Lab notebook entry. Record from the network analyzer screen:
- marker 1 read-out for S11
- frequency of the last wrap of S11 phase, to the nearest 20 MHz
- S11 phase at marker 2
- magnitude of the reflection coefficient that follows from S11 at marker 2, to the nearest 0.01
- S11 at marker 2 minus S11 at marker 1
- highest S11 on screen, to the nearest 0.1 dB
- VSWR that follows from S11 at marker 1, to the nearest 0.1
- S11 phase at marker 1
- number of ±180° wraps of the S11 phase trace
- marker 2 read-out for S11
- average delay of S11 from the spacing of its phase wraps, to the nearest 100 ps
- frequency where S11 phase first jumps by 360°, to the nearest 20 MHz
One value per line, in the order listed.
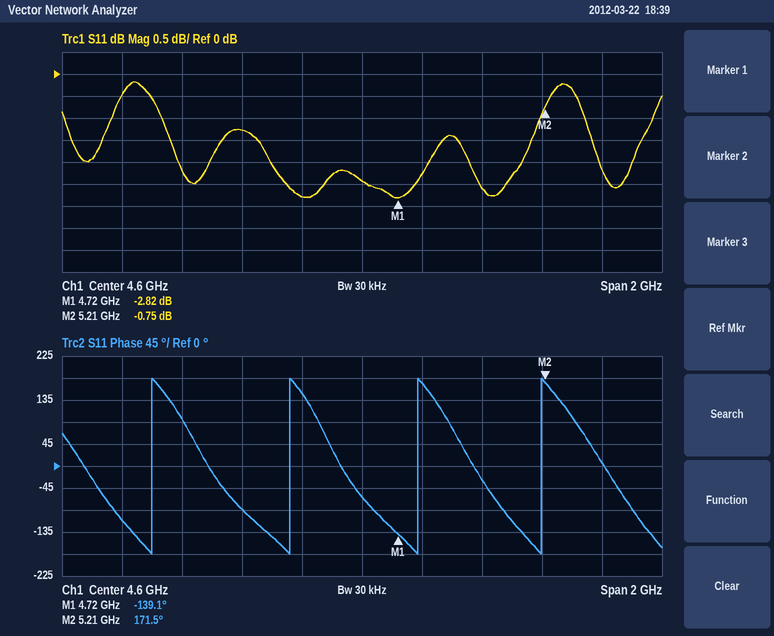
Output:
-2.82 dB
5.20 GHz
171.5°
0.92
2.07 dB
-0.2 dB
6.2
-139.1°
4
-0.75 dB
2.3 ns
3.90 GHz
